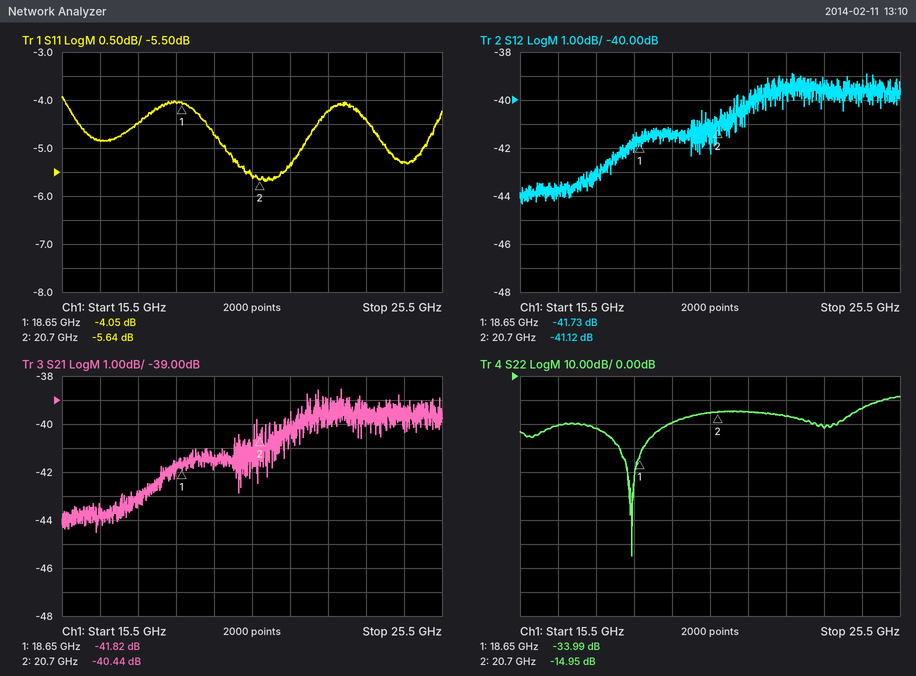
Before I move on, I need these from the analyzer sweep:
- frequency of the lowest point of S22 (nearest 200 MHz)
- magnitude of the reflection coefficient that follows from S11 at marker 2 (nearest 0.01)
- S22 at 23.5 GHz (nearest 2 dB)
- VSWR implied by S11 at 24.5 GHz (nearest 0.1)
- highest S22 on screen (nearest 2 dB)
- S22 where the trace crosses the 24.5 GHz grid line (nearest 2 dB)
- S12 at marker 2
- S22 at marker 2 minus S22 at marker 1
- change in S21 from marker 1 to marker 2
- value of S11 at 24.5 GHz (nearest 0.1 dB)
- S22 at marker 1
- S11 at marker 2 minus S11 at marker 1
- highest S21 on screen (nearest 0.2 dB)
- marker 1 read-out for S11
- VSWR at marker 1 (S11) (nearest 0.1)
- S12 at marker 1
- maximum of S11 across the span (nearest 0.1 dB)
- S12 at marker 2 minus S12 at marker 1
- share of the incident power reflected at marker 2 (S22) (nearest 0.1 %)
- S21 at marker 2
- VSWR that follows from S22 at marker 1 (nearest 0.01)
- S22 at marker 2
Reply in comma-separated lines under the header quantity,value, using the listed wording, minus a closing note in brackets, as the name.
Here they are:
quantity,value
frequency of the lowest point of S22,18.4 GHz
magnitude of the reflection coefficient that follows from S11 at marker 2,0.52
S22 at 23.5 GHz,-22 dB
VSWR implied by S11 at 24.5 GHz,3.4
highest S22 on screen,-8 dB
S22 where the trace crosses the 24.5 GHz grid line,-14 dB
S12 at marker 2,-41.12 dB
S22 at marker 2 minus S22 at marker 1,19.04 dB
change in S21 from marker 1 to marker 2,1.38 dB
value of S11 at 24.5 GHz,-5.3 dB
S22 at marker 1,-33.99 dB
S11 at marker 2 minus S11 at marker 1,-1.59 dB
highest S21 on screen,-38.6 dB
marker 1 read-out for S11,-4.05 dB
VSWR at marker 1 (S11),4.4
S12 at marker 1,-41.73 dB
maximum of S11 across the span,-3.9 dB
S12 at marker 2 minus S12 at marker 1,0.61 dB
share of the incident power reflected at marker 2 (S22),3.2 %
S21 at marker 2,-40.44 dB
VSWR that follows from S22 at marker 1,1.04
S22 at marker 2,-14.95 dB
